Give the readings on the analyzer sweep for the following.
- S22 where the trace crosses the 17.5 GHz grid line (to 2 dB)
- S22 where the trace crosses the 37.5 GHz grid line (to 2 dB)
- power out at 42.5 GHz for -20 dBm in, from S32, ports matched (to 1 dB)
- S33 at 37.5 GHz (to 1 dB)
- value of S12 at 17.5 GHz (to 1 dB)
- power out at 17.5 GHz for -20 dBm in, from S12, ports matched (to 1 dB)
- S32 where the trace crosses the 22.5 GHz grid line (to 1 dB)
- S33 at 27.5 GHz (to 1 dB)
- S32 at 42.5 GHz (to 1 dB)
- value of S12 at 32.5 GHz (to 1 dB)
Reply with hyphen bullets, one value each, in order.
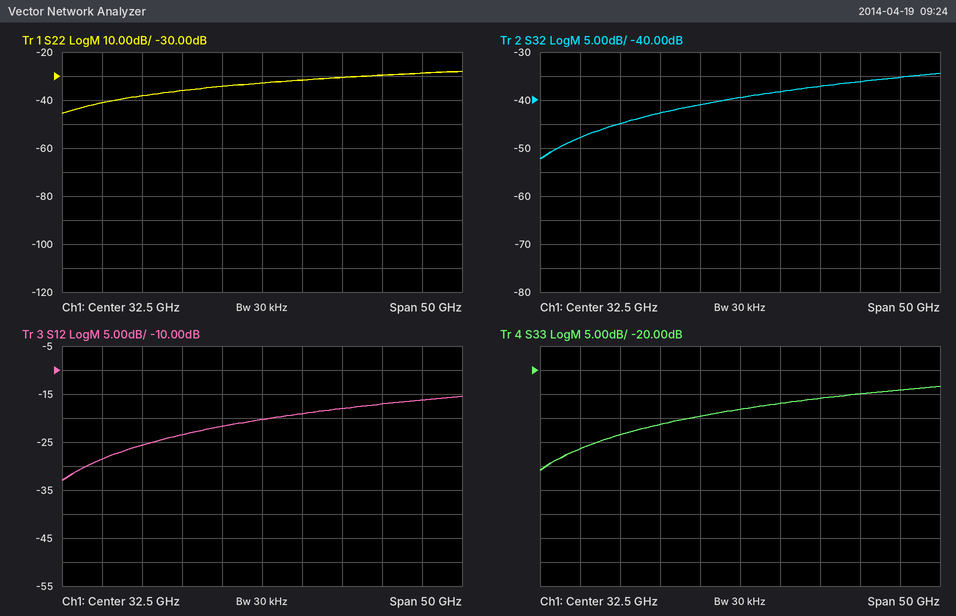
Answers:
- -38 dB
- -32 dB
- -57 dBm
- -27 dB
- -26 dB
- -46 dBm
- -43 dB
- -30 dB
- -37 dB
- -20 dB
